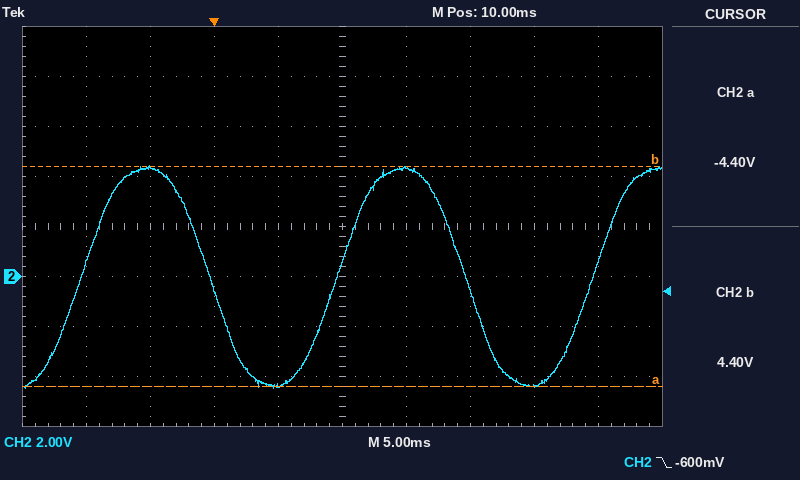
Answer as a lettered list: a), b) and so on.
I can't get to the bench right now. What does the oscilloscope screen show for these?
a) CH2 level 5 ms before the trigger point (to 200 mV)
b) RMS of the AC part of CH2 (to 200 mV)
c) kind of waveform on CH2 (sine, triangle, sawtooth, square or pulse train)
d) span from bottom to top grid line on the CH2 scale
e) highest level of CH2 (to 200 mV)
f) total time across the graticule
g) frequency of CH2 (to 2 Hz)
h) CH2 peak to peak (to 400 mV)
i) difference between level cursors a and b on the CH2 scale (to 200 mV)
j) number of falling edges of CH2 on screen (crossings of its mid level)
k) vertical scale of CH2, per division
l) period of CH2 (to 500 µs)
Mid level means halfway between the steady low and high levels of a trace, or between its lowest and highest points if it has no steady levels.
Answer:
a) 4.4 V
b) 3.2 V
c) sine
d) 16 V
e) 4.4 V
f) 50 ms
g) 50 Hz
h) 8.8 V
i) 8.8 V
j) 2
k) 2 V
l) 20.0 ms
